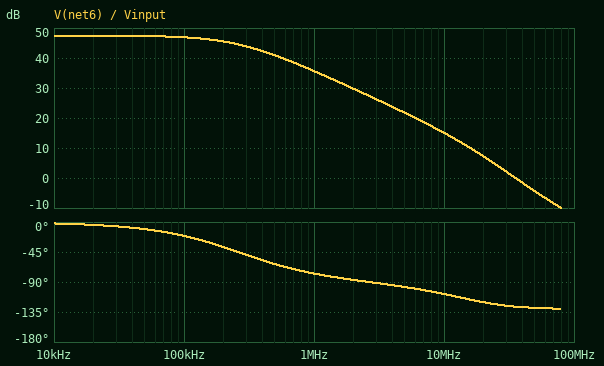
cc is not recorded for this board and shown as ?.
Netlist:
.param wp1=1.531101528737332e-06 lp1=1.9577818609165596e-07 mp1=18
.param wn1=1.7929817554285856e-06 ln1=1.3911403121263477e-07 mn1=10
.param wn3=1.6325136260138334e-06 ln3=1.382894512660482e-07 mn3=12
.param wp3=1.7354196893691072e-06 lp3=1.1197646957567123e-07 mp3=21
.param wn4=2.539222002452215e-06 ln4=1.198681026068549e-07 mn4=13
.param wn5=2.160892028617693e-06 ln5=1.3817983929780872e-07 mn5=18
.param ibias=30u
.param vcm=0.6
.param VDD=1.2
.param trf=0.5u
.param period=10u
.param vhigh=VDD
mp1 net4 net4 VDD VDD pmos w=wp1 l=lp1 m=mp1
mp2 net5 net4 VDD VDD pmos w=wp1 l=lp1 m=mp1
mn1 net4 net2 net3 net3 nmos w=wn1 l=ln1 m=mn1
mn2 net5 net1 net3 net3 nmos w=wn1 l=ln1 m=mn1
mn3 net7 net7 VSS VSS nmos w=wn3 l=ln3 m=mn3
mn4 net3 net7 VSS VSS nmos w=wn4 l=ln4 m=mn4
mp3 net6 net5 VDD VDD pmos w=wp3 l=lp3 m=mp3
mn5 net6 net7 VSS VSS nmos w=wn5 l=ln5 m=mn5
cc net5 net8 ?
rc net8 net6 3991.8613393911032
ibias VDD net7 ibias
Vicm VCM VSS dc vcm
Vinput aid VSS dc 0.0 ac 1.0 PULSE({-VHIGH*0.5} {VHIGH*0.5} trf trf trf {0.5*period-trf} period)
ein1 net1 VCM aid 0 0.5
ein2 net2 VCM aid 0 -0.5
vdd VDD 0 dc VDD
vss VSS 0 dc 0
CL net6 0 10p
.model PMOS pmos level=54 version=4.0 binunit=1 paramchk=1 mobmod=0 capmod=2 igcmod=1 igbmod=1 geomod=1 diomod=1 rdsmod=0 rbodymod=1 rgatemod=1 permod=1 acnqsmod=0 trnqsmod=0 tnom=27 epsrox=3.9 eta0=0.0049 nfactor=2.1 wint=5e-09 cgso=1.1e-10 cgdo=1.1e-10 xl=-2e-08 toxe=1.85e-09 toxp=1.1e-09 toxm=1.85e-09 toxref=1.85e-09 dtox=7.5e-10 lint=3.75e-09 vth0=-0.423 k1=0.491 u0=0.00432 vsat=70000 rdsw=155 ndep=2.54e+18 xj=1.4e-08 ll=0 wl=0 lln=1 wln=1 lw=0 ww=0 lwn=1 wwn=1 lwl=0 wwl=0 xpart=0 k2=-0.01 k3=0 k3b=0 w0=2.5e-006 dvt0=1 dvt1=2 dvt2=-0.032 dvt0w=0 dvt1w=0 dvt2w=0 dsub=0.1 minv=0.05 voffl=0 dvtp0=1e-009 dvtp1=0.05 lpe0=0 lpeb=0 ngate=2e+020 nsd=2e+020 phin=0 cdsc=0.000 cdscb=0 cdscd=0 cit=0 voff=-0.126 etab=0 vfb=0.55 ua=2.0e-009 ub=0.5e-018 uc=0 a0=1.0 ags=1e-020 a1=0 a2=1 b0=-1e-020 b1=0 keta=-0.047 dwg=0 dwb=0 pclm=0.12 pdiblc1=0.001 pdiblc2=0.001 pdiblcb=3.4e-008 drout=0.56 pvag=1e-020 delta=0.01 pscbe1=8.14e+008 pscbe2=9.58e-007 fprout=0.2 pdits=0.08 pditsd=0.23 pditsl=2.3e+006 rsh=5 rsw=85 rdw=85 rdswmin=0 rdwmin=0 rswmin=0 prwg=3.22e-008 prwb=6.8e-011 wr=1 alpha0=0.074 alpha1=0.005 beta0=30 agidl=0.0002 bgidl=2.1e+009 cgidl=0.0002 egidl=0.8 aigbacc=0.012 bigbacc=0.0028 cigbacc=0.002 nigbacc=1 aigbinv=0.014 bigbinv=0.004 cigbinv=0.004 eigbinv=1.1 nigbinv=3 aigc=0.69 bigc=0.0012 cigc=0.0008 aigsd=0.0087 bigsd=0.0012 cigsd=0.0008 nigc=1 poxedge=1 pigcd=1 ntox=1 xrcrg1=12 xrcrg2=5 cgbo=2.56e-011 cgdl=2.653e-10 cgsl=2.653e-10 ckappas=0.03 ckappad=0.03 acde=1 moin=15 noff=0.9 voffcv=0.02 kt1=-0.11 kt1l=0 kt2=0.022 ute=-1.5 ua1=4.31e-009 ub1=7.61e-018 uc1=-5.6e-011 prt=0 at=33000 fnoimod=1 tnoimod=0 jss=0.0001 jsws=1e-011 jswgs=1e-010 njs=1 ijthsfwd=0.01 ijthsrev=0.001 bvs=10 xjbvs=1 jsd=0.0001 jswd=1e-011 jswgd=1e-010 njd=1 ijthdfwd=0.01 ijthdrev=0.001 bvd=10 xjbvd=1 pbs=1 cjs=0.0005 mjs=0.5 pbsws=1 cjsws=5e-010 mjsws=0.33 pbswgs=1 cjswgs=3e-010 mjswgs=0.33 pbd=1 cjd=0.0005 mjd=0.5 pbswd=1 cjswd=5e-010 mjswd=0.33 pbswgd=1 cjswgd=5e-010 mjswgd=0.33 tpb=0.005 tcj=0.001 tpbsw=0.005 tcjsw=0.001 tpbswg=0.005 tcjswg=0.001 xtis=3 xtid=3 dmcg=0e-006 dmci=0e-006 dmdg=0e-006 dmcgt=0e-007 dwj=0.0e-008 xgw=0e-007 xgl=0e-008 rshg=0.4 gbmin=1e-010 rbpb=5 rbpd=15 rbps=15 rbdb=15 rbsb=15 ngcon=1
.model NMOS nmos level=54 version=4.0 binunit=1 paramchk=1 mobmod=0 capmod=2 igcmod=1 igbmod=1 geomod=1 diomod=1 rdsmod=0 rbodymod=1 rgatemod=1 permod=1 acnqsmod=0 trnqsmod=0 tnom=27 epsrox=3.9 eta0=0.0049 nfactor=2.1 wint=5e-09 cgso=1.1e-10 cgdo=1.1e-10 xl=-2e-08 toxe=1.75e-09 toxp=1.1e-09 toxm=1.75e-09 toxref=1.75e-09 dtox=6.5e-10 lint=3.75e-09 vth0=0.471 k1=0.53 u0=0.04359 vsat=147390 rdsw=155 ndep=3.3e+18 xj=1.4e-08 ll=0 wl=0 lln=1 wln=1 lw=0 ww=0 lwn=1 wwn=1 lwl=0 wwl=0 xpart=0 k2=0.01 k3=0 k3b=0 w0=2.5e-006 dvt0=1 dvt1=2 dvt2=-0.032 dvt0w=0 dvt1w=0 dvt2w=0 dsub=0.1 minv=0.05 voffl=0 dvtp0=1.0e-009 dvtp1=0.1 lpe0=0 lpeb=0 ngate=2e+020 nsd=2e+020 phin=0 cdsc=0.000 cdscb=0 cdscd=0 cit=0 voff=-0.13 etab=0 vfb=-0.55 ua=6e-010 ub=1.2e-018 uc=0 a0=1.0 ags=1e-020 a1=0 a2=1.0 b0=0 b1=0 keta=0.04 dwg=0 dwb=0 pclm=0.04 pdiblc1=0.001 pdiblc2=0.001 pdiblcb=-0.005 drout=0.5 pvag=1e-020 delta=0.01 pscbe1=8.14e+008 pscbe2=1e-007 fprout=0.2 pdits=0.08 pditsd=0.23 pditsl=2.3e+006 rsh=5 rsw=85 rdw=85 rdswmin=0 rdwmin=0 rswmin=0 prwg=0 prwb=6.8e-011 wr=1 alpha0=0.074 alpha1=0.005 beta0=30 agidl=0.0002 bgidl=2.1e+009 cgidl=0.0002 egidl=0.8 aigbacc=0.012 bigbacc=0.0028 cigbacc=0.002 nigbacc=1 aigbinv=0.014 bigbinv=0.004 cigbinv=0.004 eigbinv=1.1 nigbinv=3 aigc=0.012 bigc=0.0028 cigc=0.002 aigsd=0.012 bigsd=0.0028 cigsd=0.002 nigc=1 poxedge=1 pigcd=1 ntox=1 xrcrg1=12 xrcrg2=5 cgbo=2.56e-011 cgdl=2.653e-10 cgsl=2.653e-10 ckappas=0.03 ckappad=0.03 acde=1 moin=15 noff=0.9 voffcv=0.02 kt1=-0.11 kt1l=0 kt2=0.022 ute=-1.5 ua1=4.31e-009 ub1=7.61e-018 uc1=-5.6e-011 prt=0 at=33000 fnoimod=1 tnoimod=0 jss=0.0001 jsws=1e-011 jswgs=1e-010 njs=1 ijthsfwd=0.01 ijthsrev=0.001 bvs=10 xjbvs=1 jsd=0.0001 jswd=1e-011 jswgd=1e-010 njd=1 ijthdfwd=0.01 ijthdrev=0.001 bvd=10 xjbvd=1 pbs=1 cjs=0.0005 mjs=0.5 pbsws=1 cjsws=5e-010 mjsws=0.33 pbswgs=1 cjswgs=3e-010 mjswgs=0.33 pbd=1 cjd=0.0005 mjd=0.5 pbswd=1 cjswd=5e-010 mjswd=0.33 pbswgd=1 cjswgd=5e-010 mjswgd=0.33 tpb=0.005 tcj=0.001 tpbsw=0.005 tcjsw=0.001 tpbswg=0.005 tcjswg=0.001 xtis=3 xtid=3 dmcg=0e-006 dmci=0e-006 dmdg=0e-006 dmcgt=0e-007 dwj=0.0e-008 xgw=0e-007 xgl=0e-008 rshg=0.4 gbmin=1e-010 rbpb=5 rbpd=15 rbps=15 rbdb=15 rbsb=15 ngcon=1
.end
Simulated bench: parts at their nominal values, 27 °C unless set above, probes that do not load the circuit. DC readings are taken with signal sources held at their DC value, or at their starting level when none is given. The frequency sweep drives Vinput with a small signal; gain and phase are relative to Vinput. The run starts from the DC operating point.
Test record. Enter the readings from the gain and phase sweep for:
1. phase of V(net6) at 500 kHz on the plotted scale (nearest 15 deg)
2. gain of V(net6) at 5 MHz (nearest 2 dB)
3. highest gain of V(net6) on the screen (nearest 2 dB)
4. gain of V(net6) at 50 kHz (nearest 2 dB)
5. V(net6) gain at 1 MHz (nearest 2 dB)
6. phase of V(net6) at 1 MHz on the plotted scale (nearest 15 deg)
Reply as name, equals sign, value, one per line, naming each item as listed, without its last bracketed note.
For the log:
phase of V(net6) at 500 kHz on the plotted scale = -60 deg
gain of V(net6) at 5 MHz = 22 dB
highest gain of V(net6) on the screen = 48 dB
gain of V(net6) at 50 kHz = 48 dB
V(net6) gain at 1 MHz = 36 dB
phase of V(net6) at 1 MHz on the plotted scale = -75 deg
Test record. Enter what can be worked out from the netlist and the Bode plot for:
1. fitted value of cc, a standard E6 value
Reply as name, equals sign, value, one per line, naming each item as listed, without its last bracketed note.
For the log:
fitted value of cc, a standard E6 value = 1 pF
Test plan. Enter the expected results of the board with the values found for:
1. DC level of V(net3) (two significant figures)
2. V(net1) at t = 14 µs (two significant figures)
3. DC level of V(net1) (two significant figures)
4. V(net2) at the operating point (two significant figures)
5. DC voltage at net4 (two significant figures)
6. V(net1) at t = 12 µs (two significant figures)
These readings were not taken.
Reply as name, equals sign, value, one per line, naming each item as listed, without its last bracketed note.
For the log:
DC level of V(net3) = 210 mV
V(net1) at t = 14 µs = 900 mV
DC level of V(net1) = 600 mV
V(net2) at the operating point = 600 mV
DC voltage at net4 = 710 mV
V(net1) at t = 12 µs = 900 mV
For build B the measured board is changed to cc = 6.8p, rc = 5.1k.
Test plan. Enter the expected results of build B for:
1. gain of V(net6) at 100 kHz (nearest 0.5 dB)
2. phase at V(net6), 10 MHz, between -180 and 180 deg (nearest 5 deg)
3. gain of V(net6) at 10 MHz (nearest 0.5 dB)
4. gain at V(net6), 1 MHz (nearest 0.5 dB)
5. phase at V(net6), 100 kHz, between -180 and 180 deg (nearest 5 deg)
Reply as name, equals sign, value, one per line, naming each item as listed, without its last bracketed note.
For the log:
gain of V(net6) at 100 kHz = 39.0 dB
phase at V(net6), 10 MHz, between -180 and 180 deg = -60 deg
gain of V(net6) at 10 MHz = 5.0 dB
gain at V(net6), 1 MHz = 20.0 dB
phase at V(net6), 100 kHz, between -180 and 180 deg = -65 deg
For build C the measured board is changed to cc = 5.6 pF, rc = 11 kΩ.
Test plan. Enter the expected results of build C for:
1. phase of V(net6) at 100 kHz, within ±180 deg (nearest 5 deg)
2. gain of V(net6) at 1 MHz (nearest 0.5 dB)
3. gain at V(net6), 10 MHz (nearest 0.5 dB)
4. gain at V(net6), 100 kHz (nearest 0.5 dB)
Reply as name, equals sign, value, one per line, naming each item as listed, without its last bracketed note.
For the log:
phase of V(net6) at 100 kHz, within ±180 deg = -60 deg
gain of V(net6) at 1 MHz = 22.0 dB
gain at V(net6), 10 MHz = 11.5 dB
gain at V(net6), 100 kHz = 40.5 dB
